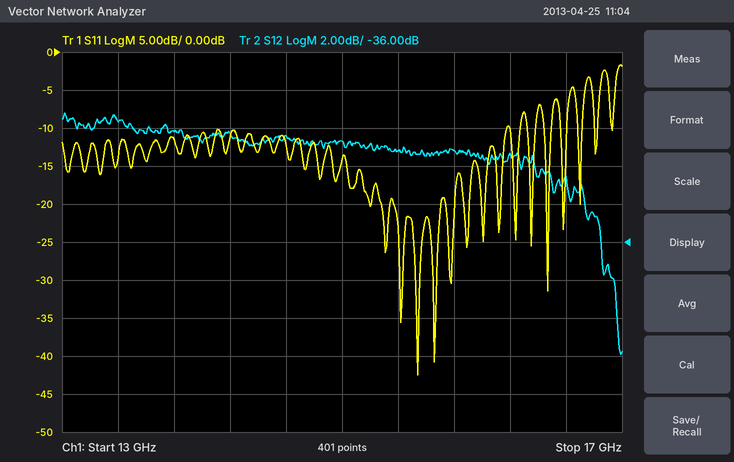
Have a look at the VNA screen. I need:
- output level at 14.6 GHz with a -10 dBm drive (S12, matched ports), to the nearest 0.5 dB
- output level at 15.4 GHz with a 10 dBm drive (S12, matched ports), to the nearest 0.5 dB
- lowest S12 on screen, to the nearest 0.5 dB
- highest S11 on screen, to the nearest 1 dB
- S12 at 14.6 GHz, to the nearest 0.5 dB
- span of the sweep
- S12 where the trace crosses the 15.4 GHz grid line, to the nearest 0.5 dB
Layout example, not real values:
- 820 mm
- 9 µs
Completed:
- -40.5 dBm
- -21.0 dBm
- -42.0 dB
- -2 dB
- -30.5 dB
- 4 GHz
- -31.0 dB
